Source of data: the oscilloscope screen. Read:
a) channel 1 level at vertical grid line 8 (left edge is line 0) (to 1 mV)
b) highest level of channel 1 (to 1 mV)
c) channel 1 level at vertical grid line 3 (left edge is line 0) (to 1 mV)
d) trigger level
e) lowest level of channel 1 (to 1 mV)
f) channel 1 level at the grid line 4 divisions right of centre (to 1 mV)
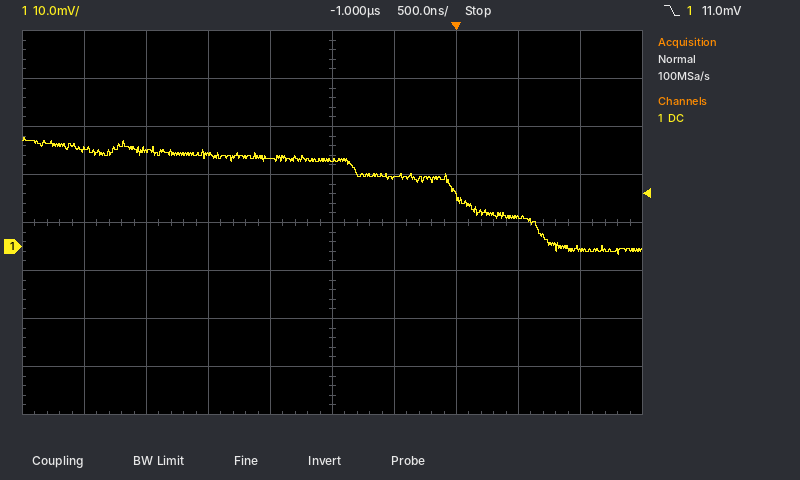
6 mV
23 mV
19 mV
11.0 mV
-2 mV
0 mV
